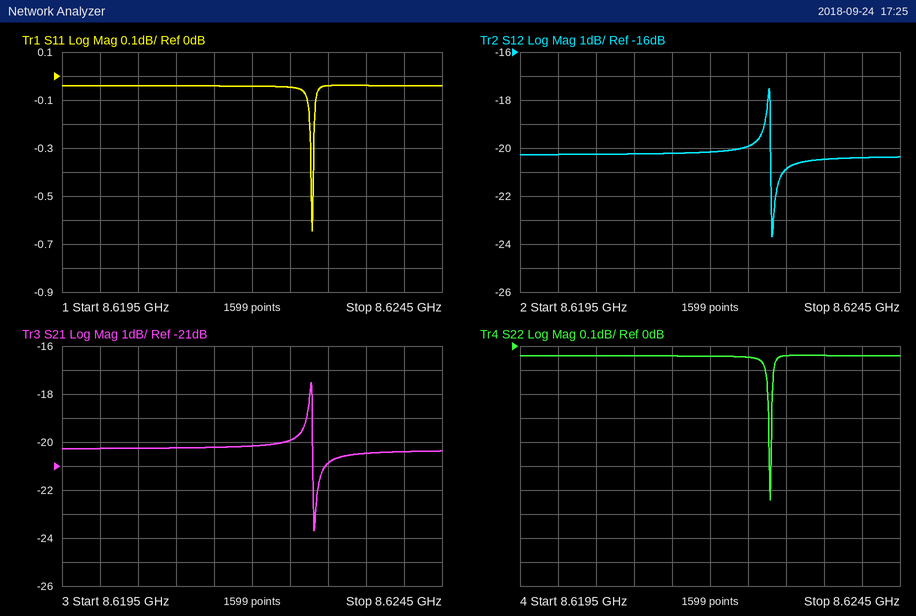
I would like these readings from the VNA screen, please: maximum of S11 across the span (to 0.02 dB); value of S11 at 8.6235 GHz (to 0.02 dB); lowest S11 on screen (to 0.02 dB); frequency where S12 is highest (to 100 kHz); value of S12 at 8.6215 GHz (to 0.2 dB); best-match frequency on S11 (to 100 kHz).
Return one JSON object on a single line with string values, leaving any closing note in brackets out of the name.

{"maximum of S11 across the span": "-0.04 dB", "value of S11 at 8.6235 GHz": "-0.04 dB", "lowest S11 on screen": "-0.64 dB", "frequency where S12 is highest": "8.6228 GHz", "value of S12 at 8.6215 GHz": "-20.2 dB", "best-match frequency on S11": "8.6228 GHz"}
